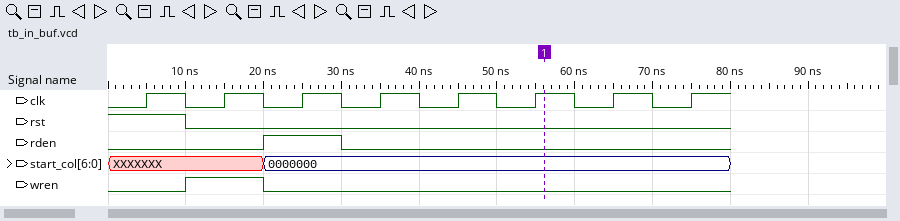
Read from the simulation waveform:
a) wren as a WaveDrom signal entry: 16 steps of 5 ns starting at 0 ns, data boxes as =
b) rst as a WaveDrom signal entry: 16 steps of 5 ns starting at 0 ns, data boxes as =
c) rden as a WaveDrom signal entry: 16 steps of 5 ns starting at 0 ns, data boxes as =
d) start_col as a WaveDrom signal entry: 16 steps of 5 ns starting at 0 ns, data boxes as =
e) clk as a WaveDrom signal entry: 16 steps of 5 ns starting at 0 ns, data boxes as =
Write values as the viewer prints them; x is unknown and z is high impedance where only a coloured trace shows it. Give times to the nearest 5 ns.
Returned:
{name: 'wren', wave: '0.1.0...........'}
{name: 'rst', wave: '1.0.............'}
{name: 'rden', wave: '0...1.0.........'}
{name: 'start_col', wave: 'x...=...........', data: '0000000'}
{name: 'clk', wave: '0101010101010101'}
